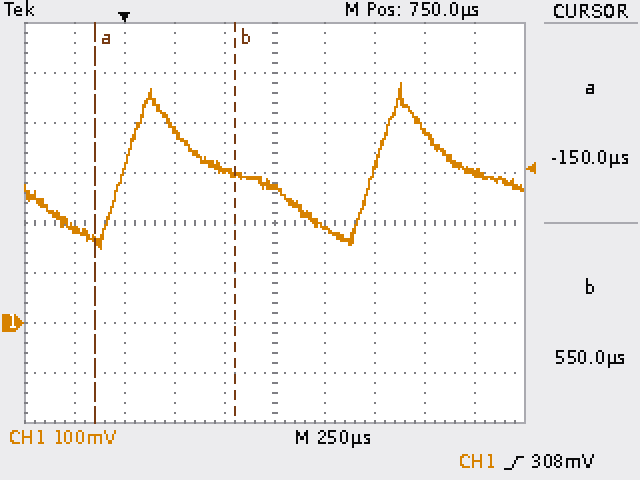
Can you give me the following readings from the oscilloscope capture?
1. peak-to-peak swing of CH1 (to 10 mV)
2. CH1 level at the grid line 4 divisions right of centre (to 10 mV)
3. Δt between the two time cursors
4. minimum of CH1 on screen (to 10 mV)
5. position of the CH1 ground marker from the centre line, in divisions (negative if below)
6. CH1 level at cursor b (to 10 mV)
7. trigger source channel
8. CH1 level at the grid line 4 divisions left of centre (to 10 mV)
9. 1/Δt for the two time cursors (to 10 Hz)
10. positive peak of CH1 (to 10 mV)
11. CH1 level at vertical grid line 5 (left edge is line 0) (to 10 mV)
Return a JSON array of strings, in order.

["330 mV", "300 mV", "700 µs", "150 mV", "-2.0 div", "300 mV", "CH1", "190 mV", "1.43 kHz", "480 mV", "270 mV"]
